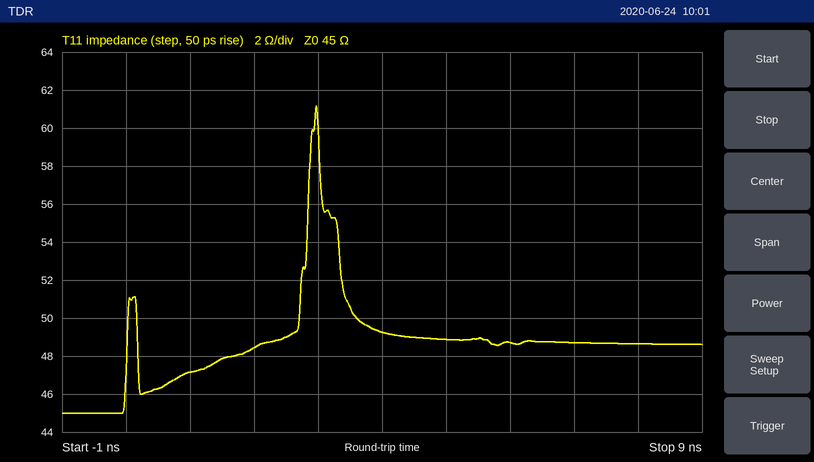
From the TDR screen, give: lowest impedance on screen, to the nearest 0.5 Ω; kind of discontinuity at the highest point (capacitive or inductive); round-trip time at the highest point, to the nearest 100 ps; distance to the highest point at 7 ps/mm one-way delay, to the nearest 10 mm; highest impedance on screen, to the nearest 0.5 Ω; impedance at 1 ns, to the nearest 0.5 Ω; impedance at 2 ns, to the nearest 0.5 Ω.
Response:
45.0 Ω
inductive
3.0 ns
210 mm
61.0 Ω
47.0 Ω
48.5 Ω
